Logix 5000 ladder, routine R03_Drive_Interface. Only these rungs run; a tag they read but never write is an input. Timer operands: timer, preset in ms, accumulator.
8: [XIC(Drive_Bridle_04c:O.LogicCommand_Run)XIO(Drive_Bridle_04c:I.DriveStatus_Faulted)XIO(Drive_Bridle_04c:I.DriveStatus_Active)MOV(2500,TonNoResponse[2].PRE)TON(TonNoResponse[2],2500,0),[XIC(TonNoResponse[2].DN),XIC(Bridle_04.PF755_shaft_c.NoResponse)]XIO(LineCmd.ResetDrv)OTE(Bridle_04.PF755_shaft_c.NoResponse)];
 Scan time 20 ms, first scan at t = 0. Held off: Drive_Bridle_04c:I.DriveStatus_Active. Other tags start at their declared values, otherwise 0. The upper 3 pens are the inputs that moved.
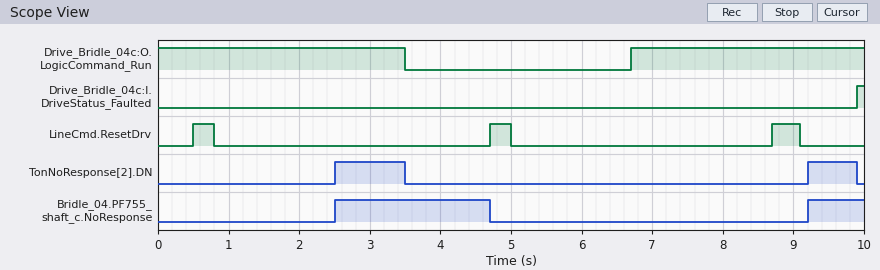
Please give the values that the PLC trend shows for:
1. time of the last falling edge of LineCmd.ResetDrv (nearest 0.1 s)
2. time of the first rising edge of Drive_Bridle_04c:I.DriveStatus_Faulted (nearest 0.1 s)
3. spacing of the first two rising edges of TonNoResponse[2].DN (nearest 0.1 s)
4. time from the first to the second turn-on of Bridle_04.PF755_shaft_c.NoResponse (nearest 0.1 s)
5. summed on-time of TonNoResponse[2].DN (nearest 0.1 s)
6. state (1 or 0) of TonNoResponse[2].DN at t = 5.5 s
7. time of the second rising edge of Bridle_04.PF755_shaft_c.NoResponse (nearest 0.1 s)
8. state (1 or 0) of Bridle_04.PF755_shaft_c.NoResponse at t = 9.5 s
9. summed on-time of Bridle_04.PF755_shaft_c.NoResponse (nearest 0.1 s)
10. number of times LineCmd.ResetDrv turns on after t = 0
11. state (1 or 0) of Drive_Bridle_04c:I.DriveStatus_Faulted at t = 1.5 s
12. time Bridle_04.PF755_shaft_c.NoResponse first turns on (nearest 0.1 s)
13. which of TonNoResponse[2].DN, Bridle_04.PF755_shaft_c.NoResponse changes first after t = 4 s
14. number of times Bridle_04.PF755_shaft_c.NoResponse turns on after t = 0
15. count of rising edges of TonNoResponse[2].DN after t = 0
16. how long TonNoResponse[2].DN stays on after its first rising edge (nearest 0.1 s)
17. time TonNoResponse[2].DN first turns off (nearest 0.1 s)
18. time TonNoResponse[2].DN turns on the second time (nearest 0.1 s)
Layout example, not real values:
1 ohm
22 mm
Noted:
9.1 s
9.9 s
6.7 s
6.7 s
1.7 s
0
9.2 s
1
3.0 s
3
0
2.5 s
Bridle_04.PF755_shaft_c.NoResponse
2
2
1.0 s
3.5 s
9.2 s
